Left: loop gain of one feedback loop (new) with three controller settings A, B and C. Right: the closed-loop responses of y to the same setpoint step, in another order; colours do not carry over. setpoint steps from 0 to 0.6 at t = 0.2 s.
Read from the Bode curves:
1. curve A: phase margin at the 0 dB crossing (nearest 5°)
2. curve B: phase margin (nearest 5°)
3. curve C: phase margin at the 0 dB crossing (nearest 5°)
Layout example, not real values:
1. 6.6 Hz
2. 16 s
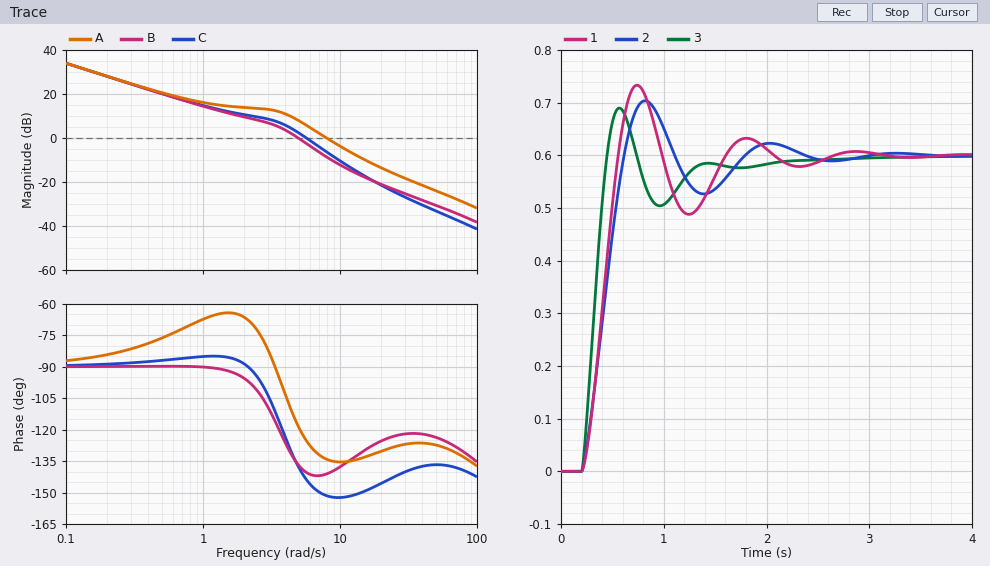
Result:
1. 45°
2. 45°
3. 35°
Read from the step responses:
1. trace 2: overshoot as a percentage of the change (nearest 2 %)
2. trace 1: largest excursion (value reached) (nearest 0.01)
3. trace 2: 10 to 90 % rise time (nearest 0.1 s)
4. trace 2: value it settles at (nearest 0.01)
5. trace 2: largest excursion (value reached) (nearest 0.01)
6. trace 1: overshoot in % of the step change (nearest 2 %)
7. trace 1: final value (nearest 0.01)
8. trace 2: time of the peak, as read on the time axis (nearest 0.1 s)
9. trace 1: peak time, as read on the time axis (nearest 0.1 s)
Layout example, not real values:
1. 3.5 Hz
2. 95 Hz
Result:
1. 18 %
2. 0.73
3. 0.3 s
4. 0.60
5. 0.70
6. 22 %
7. 0.60
8. 0.8 s
9. 0.7 s
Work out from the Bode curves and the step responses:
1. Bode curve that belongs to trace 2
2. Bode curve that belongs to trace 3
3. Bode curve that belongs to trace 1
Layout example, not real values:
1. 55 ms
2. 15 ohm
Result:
1. B
2. A
3. C
